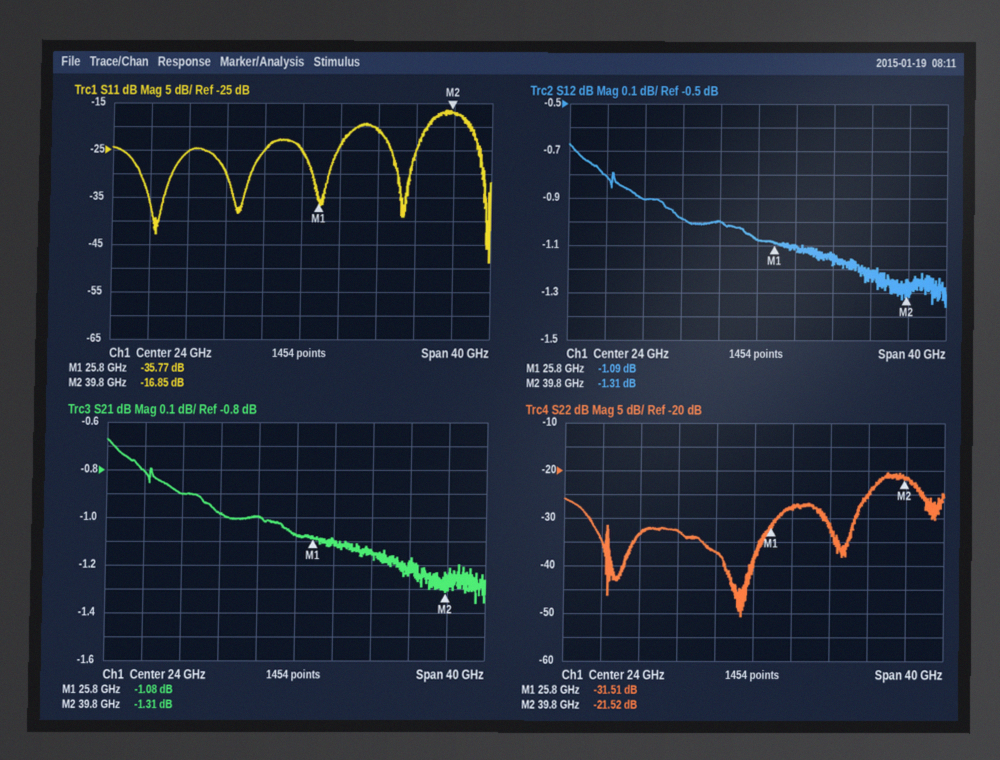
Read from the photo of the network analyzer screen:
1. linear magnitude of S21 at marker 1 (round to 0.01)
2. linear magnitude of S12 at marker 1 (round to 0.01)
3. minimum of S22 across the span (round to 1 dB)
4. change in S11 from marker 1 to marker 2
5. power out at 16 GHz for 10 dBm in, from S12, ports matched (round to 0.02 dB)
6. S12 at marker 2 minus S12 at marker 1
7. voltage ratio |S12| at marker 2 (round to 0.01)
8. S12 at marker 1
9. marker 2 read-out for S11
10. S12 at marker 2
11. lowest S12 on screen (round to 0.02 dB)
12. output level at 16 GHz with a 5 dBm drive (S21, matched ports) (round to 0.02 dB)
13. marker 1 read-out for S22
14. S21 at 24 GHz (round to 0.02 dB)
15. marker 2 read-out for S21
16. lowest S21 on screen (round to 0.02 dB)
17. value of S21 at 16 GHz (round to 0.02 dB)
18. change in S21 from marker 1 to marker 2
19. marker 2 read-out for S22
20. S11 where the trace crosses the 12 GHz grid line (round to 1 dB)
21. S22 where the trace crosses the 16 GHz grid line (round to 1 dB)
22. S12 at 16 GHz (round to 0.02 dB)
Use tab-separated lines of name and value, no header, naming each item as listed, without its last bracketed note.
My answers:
linear magnitude of S21 at marker 1	0.88
linear magnitude of S12 at marker 1	0.88
minimum of S22 across the span	-51 dB
change in S11 from marker 1 to marker 2	18.92 dB
power out at 16 GHz for 10 dBm in, from S12, ports matched	9.02 dBm
S12 at marker 2 minus S12 at marker 1	-0.22 dB
voltage ratio |S12| at marker 2	0.86
S12 at marker 1	-1.09 dB
marker 2 read-out for S11	-16.85 dB
S12 at marker 2	-1.31 dB
lowest S12 on screen	-1.36 dB
output level at 16 GHz with a 5 dBm drive (S21, matched ports)	4.02 dBm
marker 1 read-out for S22	-31.51 dB
S21 at 24 GHz	-1.08 dB
marker 2 read-out for S21	-1.31 dB
lowest S21 on screen	-1.36 dB
value of S21 at 16 GHz	-0.98 dB
change in S21 from marker 1 to marker 2	-0.23 dB
marker 2 read-out for S22	-21.52 dB
S11 where the trace crosses the 12 GHz grid line	-25 dB
S22 where the trace crosses the 16 GHz grid line	-33 dB
S12 at 16 GHz	-0.98 dB
